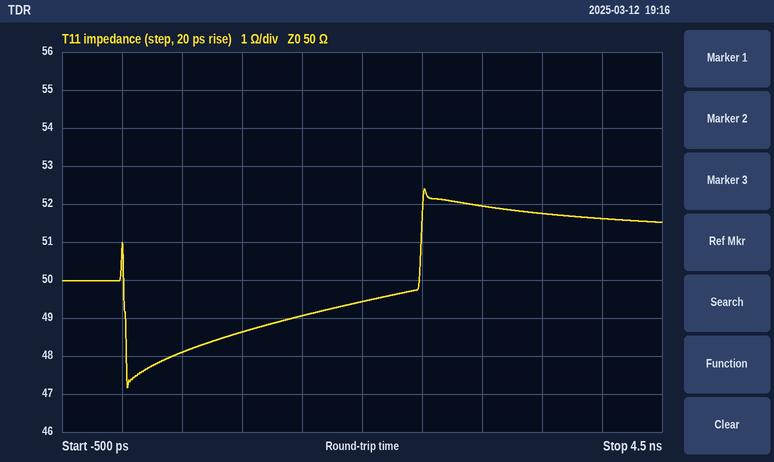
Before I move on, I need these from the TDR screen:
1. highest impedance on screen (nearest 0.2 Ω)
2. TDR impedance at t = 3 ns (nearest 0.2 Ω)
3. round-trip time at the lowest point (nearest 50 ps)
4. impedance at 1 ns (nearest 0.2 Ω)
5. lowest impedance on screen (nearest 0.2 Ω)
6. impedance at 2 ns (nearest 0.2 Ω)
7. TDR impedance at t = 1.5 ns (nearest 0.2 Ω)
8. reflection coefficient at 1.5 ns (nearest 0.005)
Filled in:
52.4 Ω
52.0 Ω
50 ps
48.6 Ω
47.2 Ω
49.4 Ω
49.0 Ω
-0.010
